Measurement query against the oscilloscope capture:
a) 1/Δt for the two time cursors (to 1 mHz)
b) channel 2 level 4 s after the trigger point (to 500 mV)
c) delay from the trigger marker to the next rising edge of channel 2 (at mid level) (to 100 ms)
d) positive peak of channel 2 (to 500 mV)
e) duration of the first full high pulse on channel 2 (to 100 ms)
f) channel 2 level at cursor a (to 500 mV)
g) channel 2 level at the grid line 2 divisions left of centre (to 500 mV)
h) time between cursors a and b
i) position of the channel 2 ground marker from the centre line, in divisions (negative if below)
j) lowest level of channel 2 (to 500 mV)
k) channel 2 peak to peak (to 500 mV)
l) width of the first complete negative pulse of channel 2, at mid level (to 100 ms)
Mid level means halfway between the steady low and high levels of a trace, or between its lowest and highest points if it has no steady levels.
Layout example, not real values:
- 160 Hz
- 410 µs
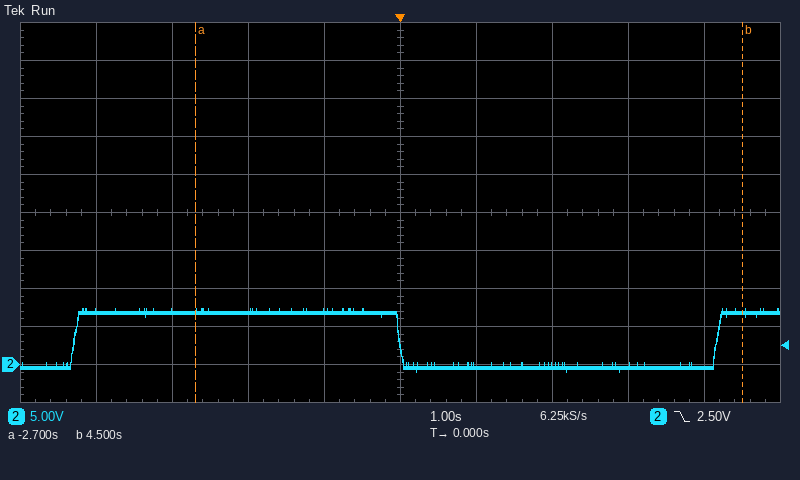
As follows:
- 139 mHz
- -500 mV
- 4.2 s
- 7.5 V
- 4.3 s
- 7.0 V
- 7.0 V
- 7.2 s
- -4.0 div
- -1.0 V
- 8.5 V
- 4.2 s
